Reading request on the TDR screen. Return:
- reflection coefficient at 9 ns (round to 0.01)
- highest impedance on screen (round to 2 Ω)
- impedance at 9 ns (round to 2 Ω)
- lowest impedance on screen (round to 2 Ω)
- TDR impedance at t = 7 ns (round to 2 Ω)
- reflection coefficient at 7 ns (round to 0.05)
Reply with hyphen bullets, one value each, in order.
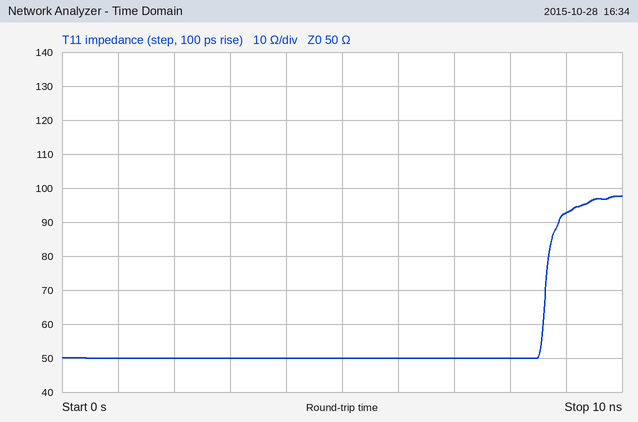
- +0.30
- 98 Ω
- 92 Ω
- 50 Ω
- 50 Ω
- 0.00
